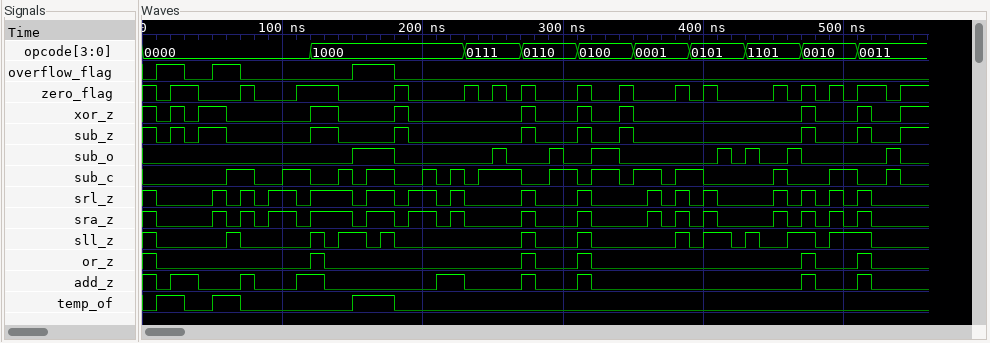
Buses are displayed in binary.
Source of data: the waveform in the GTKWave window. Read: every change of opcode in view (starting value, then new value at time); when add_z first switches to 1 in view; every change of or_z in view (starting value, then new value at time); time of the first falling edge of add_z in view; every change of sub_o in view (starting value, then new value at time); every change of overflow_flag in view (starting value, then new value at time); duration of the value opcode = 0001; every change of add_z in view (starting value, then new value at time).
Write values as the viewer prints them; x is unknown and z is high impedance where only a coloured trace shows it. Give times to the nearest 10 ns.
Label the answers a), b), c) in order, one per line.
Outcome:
a) 0000, 1000 at 120 ns, 0111 at 230 ns, 0110 at 270 ns, 0100 at 310 ns, 0001 at 350 ns, 0101 at 390 ns, 1101 at 430 ns, 0010 at 470 ns, 0011 at 510 ns
b) 20 ns
c) 1, 0 at 10 ns, 1 at 120 ns, 0 at 130 ns, 1 at 270 ns, 0 at 280 ns, 1 at 310 ns, 0 at 320 ns, 1 at 470 ns, 0 at 480 ns, 1 at 510 ns, 0 at 520 ns
d) 10 ns
e) 0, 1 at 150 ns, 0 at 180 ns, 1 at 250 ns, 0 at 260 ns, 1 at 290 ns, 0 at 300 ns, 1 at 320 ns, 0 at 340 ns, 1 at 410 ns, 0 at 420 ns, 1 at 430 ns, 0 at 440 ns, 1 at 460 ns, 0 at 470 ns, 1 at 530 ns, 0 at 540 ns
f) 0, 1 at 10 ns, 0 at 30 ns, 1 at 50 ns, 0 at 70 ns, 1 at 150 ns, 0 at 180 ns
g) 40 ns
h) 1, 0 at 10 ns, 1 at 20 ns, 0 at 40 ns, 1 at 70 ns, 0 at 80 ns, 1 at 110 ns, 0 at 130 ns, 1 at 210 ns, 0 at 230 ns, 1 at 270 ns, 0 at 280 ns, 1 at 310 ns, 0 at 320 ns, 1 at 470 ns, 0 at 480 ns, 1 at 510 ns, 0 at 520 ns
